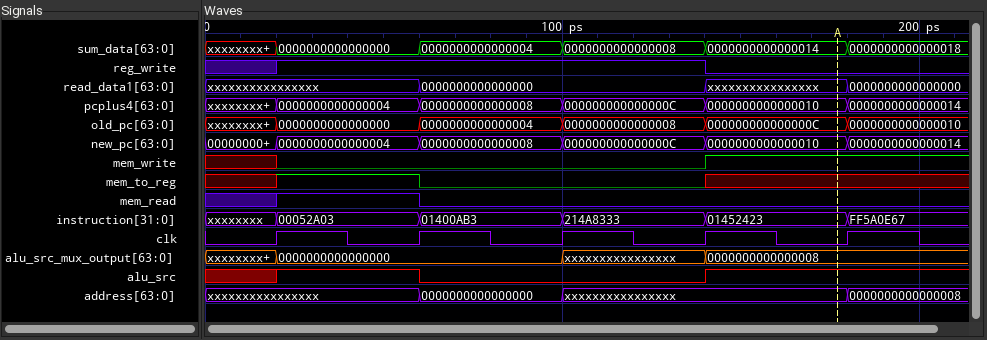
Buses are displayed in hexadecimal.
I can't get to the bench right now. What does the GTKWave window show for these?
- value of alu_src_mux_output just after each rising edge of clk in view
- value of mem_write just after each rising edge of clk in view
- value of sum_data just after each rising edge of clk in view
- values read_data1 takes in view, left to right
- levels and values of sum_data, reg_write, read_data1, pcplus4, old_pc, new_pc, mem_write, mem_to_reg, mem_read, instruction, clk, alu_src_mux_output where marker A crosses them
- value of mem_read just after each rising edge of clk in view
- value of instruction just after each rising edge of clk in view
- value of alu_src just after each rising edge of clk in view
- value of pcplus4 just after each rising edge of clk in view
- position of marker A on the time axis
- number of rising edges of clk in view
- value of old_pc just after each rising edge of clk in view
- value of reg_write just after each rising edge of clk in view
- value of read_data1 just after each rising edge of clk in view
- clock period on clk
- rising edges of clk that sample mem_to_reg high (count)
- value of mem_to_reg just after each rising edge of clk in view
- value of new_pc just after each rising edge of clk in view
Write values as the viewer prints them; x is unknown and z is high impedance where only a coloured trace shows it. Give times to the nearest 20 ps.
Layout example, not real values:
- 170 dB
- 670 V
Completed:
- 0000000000000000, 0000000000000000, xxxxxxxxxxxxxxxx, 0000000000000008, 0000000000000008
- 0 0 0 1 1
- 0000000000000000, 0000000000000004, 0000000000000008, 0000000000000014, 0000000000000018
- xxxxxxxxxxxxxxxx, 0000000000000000, xxxxxxxxxxxxxxxx, 0000000000000000
- sum_data=0000000000000014, reg_write=0, read_data1=xxxxxxxxxxxxxxxx, pcplus4=0000000000000010, old_pc=000000000000000C, new_pc=0000000000000010, mem_write=1, mem_to_reg=x, mem_read=0, instruction=01452423, clk=0, alu_src_mux_output=0000000000000008
- 1 0 0 0 0
- 00052A03, 01400AB3, 214A8333, 01452423, FF5A0E67
- 1 0 0 1 1
- 0000000000000004, 0000000000000008, 000000000000000C, 0000000000000010, 0000000000000014
- 180 ps
- 5
- 0000000000000000, 0000000000000004, 0000000000000008, 000000000000000C, 0000000000000010
- 1 1 1 0 0
- xxxxxxxxxxxxxxxx, 0000000000000000, 0000000000000000, xxxxxxxxxxxxxxxx, 0000000000000000
- 40 ps
- 1
- 1 0 0 x x
- 0000000000000004, 0000000000000008, 000000000000000C, 0000000000000010, 0000000000000014
